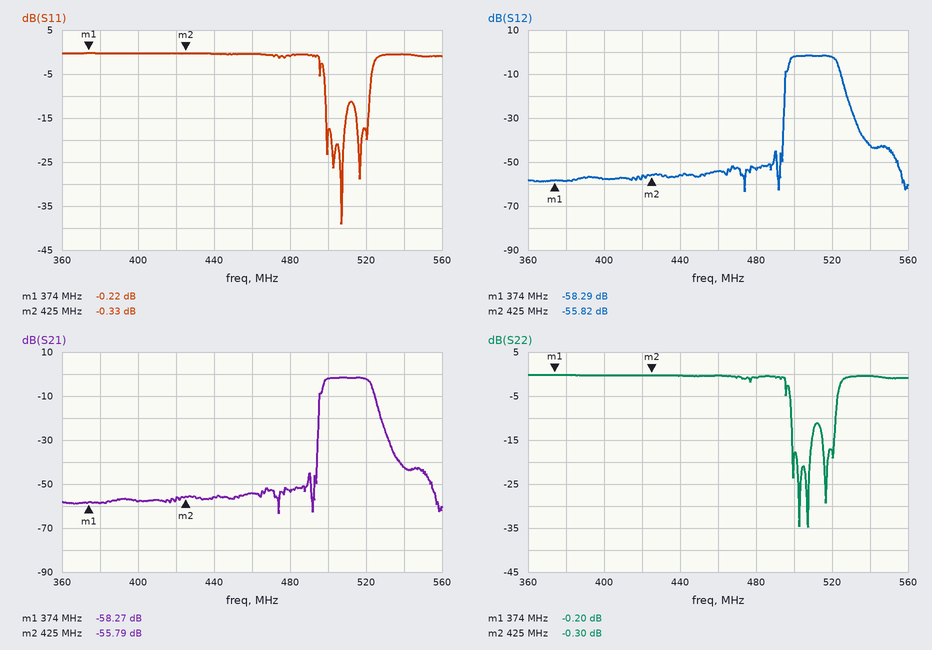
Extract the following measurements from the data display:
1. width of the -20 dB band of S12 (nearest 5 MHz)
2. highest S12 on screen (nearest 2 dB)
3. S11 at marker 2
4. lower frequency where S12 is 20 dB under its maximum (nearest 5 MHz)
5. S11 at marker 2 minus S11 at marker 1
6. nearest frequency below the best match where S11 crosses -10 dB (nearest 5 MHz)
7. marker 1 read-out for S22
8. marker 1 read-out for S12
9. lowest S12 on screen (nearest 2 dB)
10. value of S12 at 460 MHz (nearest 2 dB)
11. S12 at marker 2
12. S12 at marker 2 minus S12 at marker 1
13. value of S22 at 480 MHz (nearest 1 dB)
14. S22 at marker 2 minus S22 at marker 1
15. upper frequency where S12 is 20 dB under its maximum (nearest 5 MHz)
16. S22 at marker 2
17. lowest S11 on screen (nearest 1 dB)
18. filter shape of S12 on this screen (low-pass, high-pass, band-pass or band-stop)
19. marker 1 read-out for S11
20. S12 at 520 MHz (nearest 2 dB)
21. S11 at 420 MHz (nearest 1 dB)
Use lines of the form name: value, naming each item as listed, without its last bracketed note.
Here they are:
width of the -20 dB band of S12: 35 MHz
highest S12 on screen: -2 dB
S11 at marker 2: -0.33 dB
lower frequency where S12 is 20 dB under its maximum: 495 MHz
S11 at marker 2 minus S11 at marker 1: -0.11 dB
nearest frequency below the best match where S11 crosses -10 dB: 500 MHz
marker 1 read-out for S22: -0.20 dB
marker 1 read-out for S12: -58.29 dB
lowest S12 on screen: -64 dB
value of S12 at 460 MHz: -54 dB
S12 at marker 2: -55.82 dB
S12 at marker 2 minus S12 at marker 1: 2.47 dB
value of S22 at 480 MHz: -1 dB
S22 at marker 2 minus S22 at marker 1: -0.10 dB
upper frequency where S12 is 20 dB under its maximum: 530 MHz
S22 at marker 2: -0.30 dB
lowest S11 on screen: -39 dB
filter shape of S12 on this screen: band-pass
marker 1 read-out for S11: -0.22 dB
S12 at 520 MHz: -2 dB
S11 at 420 MHz: 0 dB
